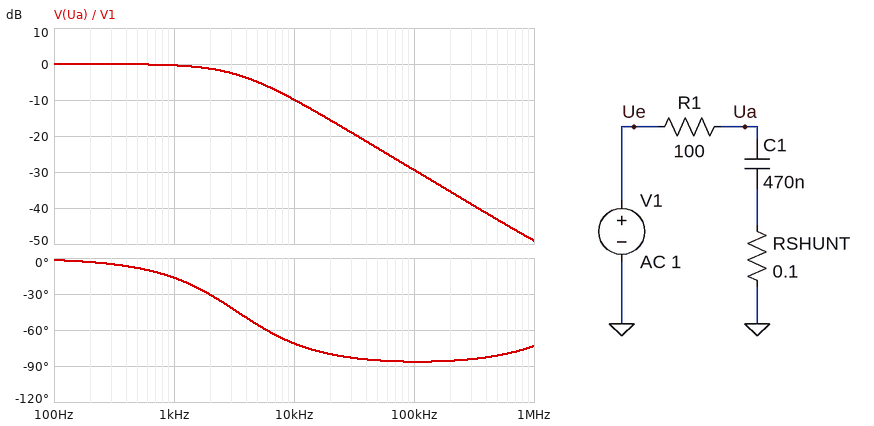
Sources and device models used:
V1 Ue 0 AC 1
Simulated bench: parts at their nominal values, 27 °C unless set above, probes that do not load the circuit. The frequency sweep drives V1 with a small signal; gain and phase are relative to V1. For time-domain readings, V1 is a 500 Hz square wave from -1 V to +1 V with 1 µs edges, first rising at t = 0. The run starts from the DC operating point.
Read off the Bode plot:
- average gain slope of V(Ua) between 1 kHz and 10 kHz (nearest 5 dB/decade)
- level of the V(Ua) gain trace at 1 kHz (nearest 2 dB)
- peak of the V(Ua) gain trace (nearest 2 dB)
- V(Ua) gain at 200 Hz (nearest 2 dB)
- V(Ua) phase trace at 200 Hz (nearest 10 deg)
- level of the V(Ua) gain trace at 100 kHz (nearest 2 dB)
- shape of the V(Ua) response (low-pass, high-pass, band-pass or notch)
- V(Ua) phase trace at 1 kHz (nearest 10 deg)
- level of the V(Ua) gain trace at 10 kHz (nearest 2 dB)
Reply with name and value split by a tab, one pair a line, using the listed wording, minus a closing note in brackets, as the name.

average gain slope of V(Ua) between 1 kHz and 10 kHz	-10 dB/decade
level of the V(Ua) gain trace at 1 kHz	0 dB
peak of the V(Ua) gain trace	0 dB
V(Ua) gain at 200 Hz	0 dB
V(Ua) phase trace at 200 Hz	0 deg
level of the V(Ua) gain trace at 100 kHz	-30 dB
shape of the V(Ua) response	low-pass
V(Ua) phase trace at 1 kHz	-20 deg
level of the V(Ua) gain trace at 10 kHz	-10 dB
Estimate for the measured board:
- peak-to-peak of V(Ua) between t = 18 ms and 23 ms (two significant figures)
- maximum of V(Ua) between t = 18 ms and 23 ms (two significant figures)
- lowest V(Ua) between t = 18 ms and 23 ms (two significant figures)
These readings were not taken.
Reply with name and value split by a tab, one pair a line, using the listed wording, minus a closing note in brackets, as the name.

peak-to-peak of V(Ua) between t = 18 ms and 23 ms	2.0 V
maximum of V(Ua) between t = 18 ms and 23 ms	1.0 V
lowest V(Ua) between t = 18 ms and 23 ms	-1.0 V
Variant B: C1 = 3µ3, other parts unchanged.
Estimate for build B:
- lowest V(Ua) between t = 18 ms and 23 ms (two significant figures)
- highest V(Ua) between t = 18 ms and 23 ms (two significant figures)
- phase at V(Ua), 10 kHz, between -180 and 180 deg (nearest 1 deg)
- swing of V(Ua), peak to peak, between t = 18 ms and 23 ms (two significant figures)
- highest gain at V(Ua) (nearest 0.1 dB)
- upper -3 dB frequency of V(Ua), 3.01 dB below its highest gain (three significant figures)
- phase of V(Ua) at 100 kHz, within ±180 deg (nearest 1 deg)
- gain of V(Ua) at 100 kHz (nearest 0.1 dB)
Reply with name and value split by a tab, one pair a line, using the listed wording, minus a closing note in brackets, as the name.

lowest V(Ua) between t = 18 ms and 23 ms	-910 mV
highest V(Ua) between t = 18 ms and 23 ms	910 mV
phase at V(Ua), 10 kHz, between -180 and 180 deg	-86 deg
swing of V(Ua), peak to peak, between t = 18 ms and 23 ms	1.8 V
highest gain at V(Ua)	0 dB
upper -3 dB frequency of V(Ua), 3.01 dB below its highest gain	482 Hz
phase of V(Ua) at 100 kHz, within ±180 deg	-78 deg
gain of V(Ua) at 100 kHz	-46.2 dB
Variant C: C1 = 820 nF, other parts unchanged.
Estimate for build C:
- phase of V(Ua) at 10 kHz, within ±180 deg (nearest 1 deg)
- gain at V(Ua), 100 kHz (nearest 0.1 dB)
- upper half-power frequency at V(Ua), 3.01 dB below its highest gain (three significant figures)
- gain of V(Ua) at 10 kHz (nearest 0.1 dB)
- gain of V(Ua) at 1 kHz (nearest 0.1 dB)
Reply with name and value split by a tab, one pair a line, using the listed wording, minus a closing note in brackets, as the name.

phase of V(Ua) at 10 kHz, within ±180 deg	-79 deg
gain at V(Ua), 100 kHz	-34.2 dB
upper half-power frequency at V(Ua), 3.01 dB below its highest gain	1.94 kHz
gain of V(Ua) at 10 kHz	-14.4 dB
gain of V(Ua) at 1 kHz	-1.0 dB
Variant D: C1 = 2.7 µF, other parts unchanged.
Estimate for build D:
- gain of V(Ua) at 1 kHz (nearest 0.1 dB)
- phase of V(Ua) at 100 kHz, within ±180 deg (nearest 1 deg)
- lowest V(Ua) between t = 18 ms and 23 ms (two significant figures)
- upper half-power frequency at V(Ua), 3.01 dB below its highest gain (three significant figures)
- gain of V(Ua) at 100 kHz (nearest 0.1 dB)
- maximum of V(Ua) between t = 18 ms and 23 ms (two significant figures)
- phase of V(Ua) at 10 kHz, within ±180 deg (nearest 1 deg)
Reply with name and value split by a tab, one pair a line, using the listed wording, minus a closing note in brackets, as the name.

gain of V(Ua) at 1 kHz	-5.9 dB
phase of V(Ua) at 100 kHz, within ±180 deg	-80 deg
lowest V(Ua) between t = 18 ms and 23 ms	-950 mV
upper half-power frequency at V(Ua), 3.01 dB below its highest gain	589 Hz
gain of V(Ua) at 100 kHz	-44.5 dB
maximum of V(Ua) between t = 18 ms and 23 ms	950 mV
phase of V(Ua) at 10 kHz, within ±180 deg	-86 deg
